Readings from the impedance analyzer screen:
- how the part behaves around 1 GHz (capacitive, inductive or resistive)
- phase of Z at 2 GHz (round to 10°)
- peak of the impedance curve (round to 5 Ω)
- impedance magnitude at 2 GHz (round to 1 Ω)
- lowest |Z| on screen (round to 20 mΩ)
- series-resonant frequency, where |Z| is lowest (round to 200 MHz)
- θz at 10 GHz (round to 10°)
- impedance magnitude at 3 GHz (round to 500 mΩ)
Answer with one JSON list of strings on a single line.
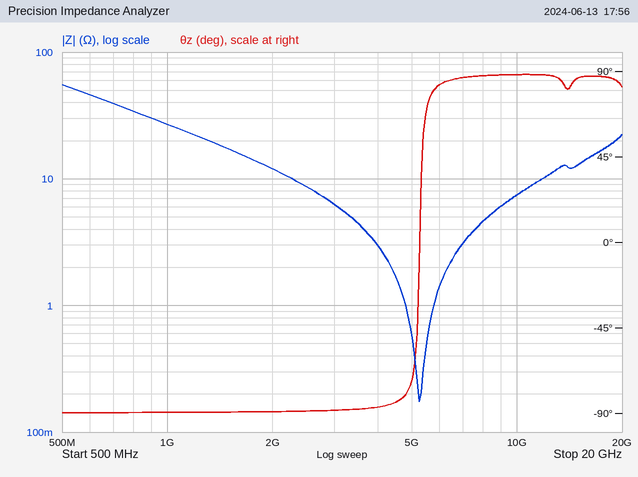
["capacitive", "-90°", "55 Ω", "12 Ω", "180 mΩ", "5.2 GHz", "90°", "6.5 Ω"]
